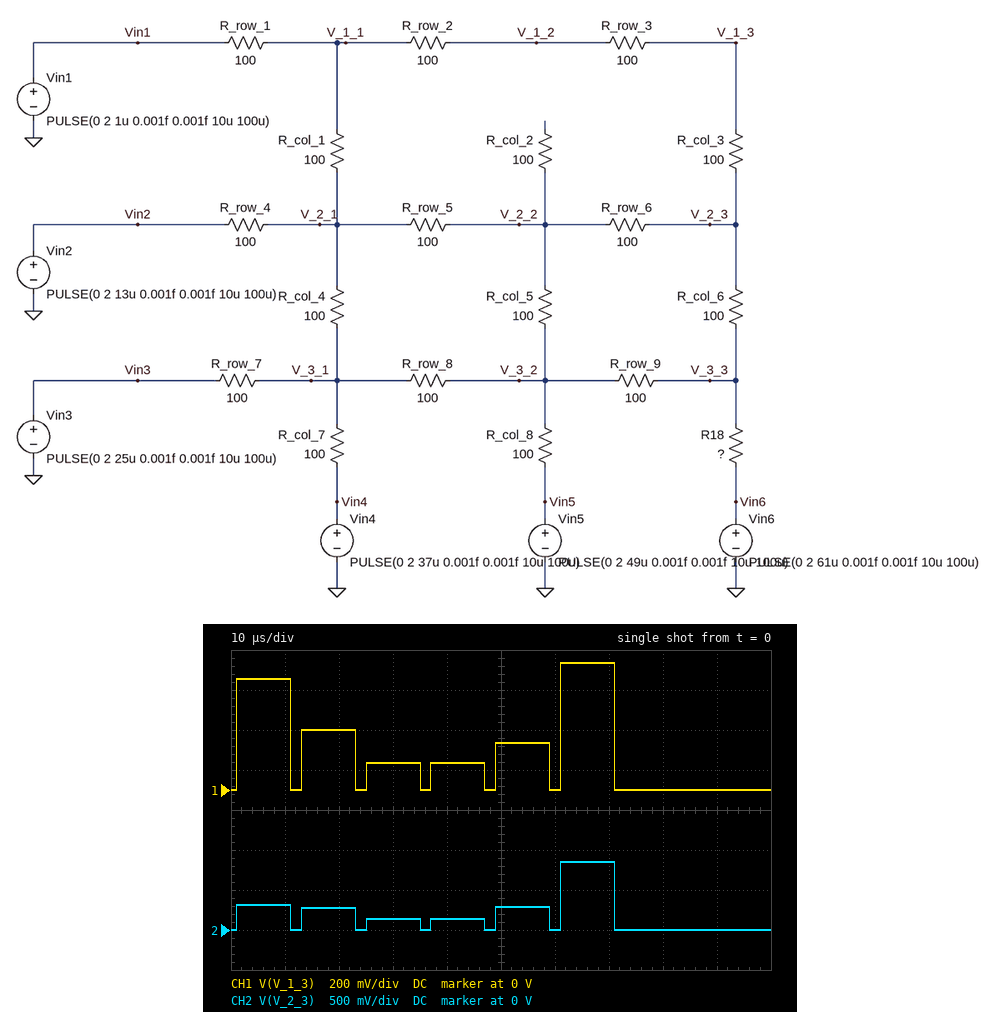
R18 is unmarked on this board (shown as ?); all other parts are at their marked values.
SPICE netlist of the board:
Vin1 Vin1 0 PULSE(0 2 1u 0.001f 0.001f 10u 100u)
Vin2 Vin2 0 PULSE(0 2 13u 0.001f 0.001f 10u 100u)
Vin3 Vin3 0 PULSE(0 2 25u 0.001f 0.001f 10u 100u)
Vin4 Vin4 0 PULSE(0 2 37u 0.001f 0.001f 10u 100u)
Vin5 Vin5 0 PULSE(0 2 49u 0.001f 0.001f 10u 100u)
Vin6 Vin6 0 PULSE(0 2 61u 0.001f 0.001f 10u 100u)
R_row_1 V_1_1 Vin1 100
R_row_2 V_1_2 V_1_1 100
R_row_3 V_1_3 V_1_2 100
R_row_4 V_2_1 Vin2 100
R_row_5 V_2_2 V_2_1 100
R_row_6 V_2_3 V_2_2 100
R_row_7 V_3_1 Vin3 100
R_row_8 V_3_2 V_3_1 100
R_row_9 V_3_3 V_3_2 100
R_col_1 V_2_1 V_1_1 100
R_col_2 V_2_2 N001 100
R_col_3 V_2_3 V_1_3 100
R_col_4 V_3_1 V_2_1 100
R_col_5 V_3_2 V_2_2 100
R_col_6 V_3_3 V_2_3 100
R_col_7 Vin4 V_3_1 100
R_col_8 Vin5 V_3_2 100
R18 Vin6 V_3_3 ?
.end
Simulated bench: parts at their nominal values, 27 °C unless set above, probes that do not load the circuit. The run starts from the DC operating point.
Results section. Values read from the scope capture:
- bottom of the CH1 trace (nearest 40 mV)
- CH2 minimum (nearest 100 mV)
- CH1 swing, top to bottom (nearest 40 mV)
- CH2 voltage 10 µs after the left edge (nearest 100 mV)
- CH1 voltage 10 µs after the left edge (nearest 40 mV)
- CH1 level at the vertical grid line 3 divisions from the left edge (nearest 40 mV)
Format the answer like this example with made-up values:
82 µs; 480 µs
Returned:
0 V; 0 V; 640 mV; 300 mV; 560 mV; 120 mV
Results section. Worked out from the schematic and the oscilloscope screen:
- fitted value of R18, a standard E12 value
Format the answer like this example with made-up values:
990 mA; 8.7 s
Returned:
47 Ω
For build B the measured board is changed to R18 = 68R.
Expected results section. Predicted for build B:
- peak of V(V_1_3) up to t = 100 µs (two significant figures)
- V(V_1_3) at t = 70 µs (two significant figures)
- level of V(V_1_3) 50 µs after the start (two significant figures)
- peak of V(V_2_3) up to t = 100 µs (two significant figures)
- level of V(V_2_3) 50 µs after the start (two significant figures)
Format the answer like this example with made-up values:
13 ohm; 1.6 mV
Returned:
570 mV; 560 mV; 270 mV; 740 mV; 330 mV
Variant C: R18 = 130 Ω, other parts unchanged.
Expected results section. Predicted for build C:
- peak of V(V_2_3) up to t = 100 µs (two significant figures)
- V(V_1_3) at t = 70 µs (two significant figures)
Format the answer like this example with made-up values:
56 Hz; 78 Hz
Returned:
540 mV; 410 mV
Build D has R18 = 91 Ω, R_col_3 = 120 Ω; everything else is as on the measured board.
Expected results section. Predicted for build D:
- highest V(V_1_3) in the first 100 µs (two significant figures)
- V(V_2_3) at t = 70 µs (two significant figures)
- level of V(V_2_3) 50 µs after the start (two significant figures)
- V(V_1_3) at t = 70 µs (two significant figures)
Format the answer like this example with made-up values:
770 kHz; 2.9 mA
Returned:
610 mV; 660 mV; 370 mV; 470 mV
